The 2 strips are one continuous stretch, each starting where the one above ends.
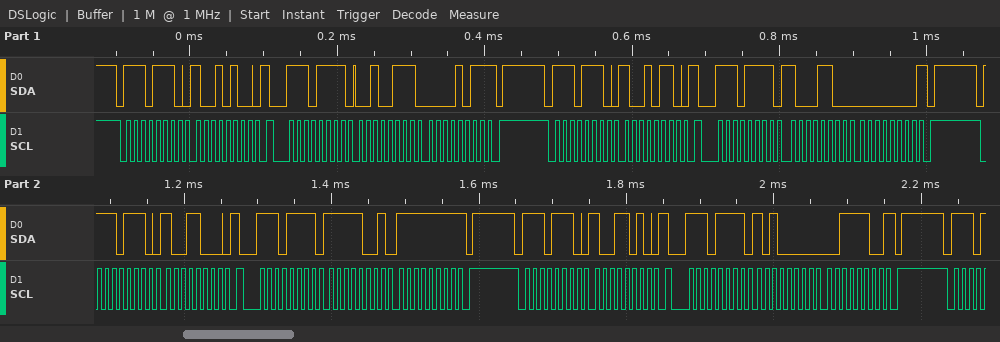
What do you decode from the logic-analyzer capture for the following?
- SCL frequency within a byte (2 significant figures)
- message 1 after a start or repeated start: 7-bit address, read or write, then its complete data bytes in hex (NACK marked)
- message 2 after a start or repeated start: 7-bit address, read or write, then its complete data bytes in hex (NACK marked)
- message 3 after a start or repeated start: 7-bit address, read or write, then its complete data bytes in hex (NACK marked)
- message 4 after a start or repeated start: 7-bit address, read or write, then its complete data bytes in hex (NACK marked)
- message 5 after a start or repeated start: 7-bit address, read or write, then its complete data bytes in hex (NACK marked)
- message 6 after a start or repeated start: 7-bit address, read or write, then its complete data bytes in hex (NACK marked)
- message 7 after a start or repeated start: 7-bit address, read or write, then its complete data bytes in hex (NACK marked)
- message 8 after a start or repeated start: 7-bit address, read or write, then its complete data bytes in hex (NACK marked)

100 kHz
0x77 write: 94
0x77 read: 27 0B NACK
0x77 write: 96
0x77 read: 8C 00 NACK
0x77 write: 98
0x77 read: F9 FF NACK
0x77 write: 9A
0x77 read: A0 3C NACK
